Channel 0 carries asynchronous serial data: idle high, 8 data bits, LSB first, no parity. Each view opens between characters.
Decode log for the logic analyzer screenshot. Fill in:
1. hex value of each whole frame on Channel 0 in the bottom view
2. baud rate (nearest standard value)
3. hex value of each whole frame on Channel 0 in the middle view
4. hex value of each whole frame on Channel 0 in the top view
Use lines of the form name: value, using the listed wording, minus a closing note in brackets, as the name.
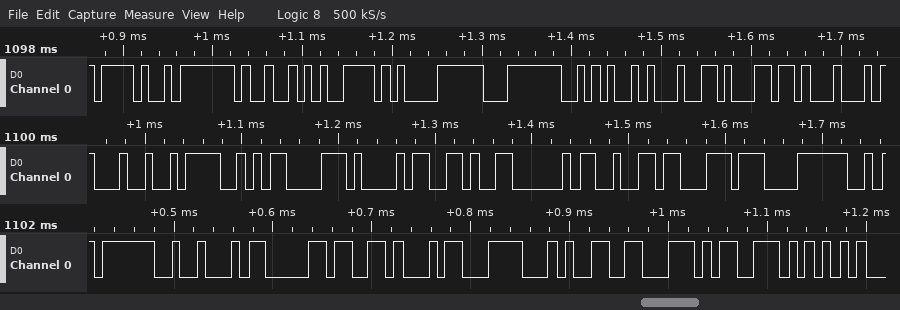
hex value of each whole frame on Channel 0 in the bottom view: 3F, A2, B0, 16, E3, 94, C6, CD, 55
baud rate: 115200 baud
hex value of each whole frame on Channel 0 in the middle view: 24, 4F, C3, A1, 96, A0, B2, DC, F8
hex value of each whole frame on Channel 0 in the top view: 2F, 7F, 52, 5E, F8, FC, 2A, 91, B1, 11
